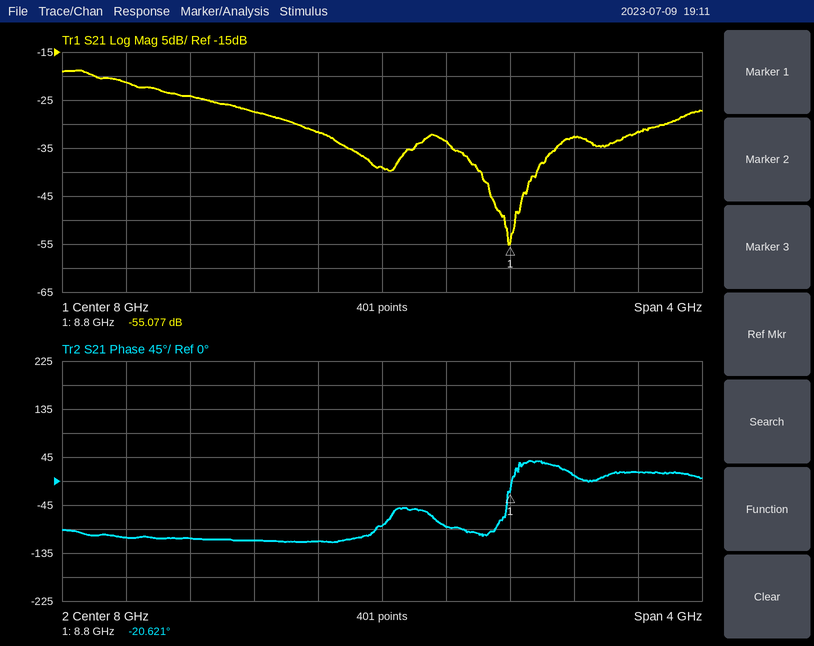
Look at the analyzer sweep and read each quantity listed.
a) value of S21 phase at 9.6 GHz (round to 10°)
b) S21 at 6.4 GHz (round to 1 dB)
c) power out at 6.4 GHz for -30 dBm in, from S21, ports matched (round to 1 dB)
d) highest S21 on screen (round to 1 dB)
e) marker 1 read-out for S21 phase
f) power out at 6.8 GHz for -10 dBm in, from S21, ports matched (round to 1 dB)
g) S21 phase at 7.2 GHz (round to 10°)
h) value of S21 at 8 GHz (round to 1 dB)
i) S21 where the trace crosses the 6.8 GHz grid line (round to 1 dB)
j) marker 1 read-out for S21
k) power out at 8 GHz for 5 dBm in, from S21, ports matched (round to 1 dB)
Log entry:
20°
-21 dB
-51 dBm
-19 dB
-20.621°
-34 dBm
-110°
-39 dB
-24 dB
-55.077 dB
-34 dBm
